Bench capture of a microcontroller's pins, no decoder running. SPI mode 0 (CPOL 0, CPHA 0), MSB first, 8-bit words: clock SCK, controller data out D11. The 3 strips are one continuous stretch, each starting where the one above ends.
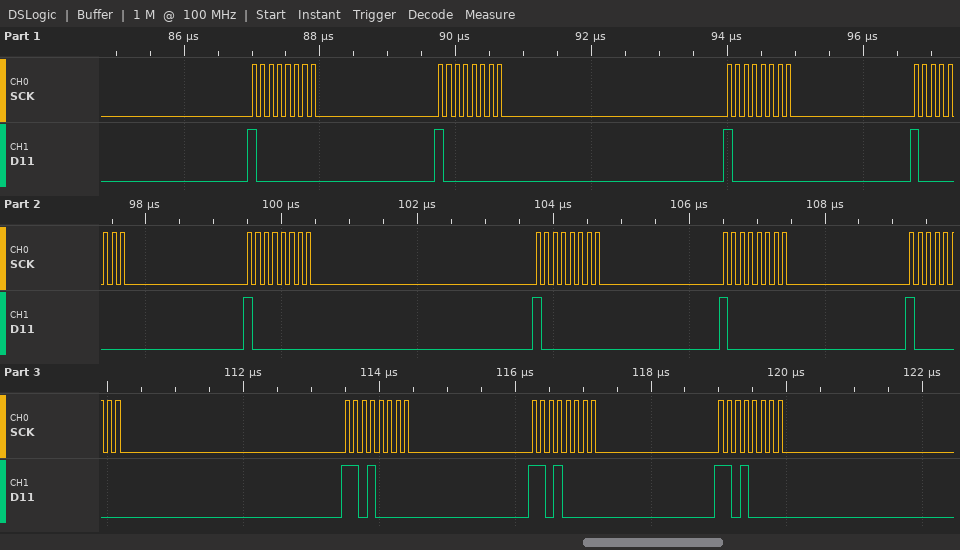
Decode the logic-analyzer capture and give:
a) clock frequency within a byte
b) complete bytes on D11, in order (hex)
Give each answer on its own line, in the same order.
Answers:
8 MHz
80 80 80 80 80 80 80 80 D0 D0 D0
